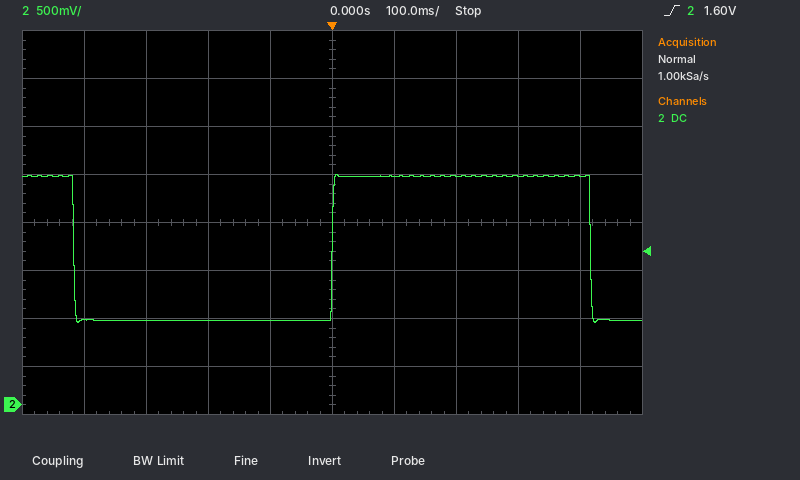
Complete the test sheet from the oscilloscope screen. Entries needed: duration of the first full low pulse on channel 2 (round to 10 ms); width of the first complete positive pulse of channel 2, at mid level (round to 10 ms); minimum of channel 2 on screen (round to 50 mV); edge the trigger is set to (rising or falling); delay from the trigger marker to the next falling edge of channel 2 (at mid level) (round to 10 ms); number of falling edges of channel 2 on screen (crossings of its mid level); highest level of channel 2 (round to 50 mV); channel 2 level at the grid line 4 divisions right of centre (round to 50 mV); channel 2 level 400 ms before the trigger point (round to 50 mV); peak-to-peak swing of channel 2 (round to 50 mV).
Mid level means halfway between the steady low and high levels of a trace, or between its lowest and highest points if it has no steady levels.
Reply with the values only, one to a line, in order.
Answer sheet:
420 ms
420 ms
850 mV
rising
420 ms
2
2.40 V
2.40 V
900 mV
1.55 V
